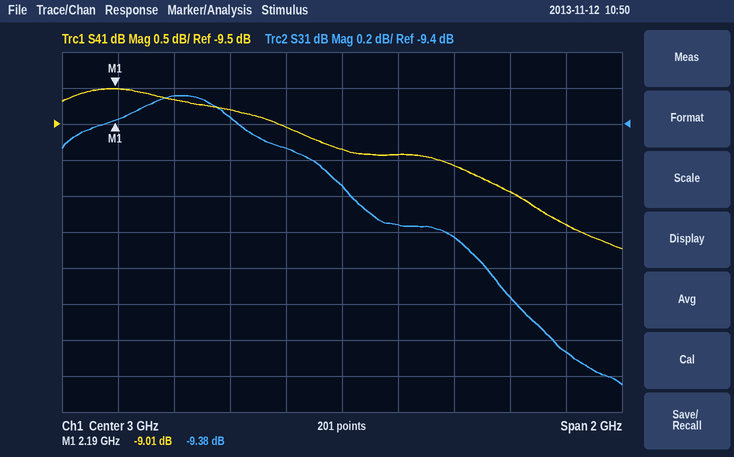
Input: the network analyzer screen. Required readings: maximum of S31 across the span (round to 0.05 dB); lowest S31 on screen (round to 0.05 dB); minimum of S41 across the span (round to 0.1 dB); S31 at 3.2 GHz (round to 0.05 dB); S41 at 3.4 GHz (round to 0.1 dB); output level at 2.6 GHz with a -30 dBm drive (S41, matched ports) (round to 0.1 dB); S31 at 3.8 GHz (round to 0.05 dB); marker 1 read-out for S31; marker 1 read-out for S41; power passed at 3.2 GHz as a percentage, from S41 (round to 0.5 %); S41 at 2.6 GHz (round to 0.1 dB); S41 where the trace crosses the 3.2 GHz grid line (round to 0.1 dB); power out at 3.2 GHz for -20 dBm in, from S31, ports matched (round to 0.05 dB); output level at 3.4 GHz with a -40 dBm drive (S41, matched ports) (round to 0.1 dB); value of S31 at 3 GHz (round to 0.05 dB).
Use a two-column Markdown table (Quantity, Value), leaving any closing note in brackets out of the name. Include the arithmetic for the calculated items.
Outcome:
| Quantity | Value |
|---|---|
| maximum of S31 across the span | -9.25 dB |
| lowest S31 on screen | -10.85 dB |
| minimum of S41 across the span | -11.2 dB |
| S31 at 3.2 GHz | -9.95 dB |
| S41 at 3.4 GHz | -10.1 dB |
| output level at 2.6 GHz with a -30 dBm drive (S41, matched ports) | -30 dBm + (-9.3 dB) = -39.3 dBm |
| S31 at 3.8 GHz | -10.65 dB |
| marker 1 read-out for S31 | -9.38 dB |
| marker 1 read-out for S41 | -9.01 dB |
| power passed at 3.2 GHz as a percentage, from S41 | 10^(-9.9/10) ≈ 10.2 %, so 10.0 % to the nearest 0.5 % |
| S41 at 2.6 GHz | -9.3 dB |
| S41 where the trace crosses the 3.2 GHz grid line | -9.9 dB |
| power out at 3.2 GHz for -20 dBm in, from S31, ports matched | -20 dBm + (-9.95 dB) = -29.95 dBm |
| output level at 3.4 GHz with a -40 dBm drive (S41, matched ports) | -40 dBm + (-10.1 dB) = -50.1 dBm |
| value of S31 at 3 GHz | -9.75 dB |
